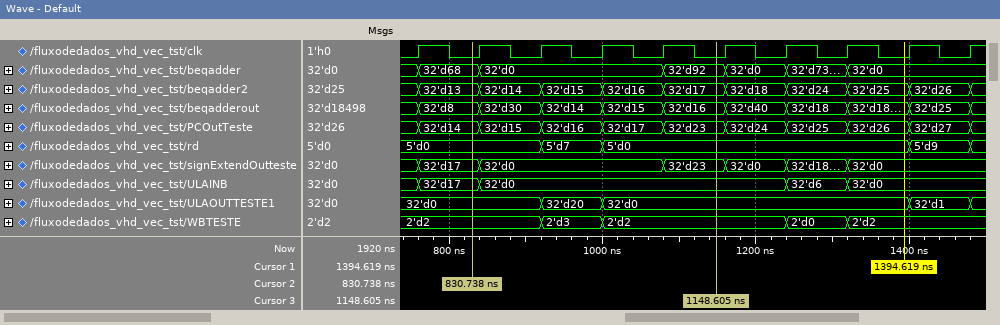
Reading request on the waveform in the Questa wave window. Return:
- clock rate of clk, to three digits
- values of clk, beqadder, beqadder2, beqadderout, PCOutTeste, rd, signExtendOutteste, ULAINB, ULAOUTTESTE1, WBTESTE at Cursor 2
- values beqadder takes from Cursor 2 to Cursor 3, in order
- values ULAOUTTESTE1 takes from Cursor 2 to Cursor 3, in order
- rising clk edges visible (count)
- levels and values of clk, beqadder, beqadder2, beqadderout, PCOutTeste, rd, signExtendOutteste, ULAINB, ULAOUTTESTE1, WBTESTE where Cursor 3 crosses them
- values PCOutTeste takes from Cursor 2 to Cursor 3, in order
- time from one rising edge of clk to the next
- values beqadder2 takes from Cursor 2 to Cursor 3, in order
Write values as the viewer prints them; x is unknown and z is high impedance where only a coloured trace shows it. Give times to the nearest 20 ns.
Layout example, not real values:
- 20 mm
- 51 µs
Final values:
- 12.5 MHz
- clk=0, beqadder=32'd68, beqadder2=32'd13, beqadderout=32'd8, PCOutTeste=32'd14, rd=5'd0, signExtendOutteste=32'd17, ULAINB=32'd17, ULAOUTTESTE1=32'd0, WBTESTE=2'd2
- 32'd68, 32'd0, 32'd92
- 32'd0, 32'd20, 32'd0
- 10
- clk=0, beqadder=32'd92, beqadder2=32'd17, beqadderout=32'd16, PCOutTeste=32'd23, rd=5'd0, signExtendOutteste=32'd23, ULAINB=32'd0, ULAOUTTESTE1=32'd0, WBTESTE=2'd2
- 32'd14, 32'd15, 32'd16, 32'd17, 32'd23
- 80 ns
- 32'd13, 32'd14, 32'd15, 32'd16, 32'd17
